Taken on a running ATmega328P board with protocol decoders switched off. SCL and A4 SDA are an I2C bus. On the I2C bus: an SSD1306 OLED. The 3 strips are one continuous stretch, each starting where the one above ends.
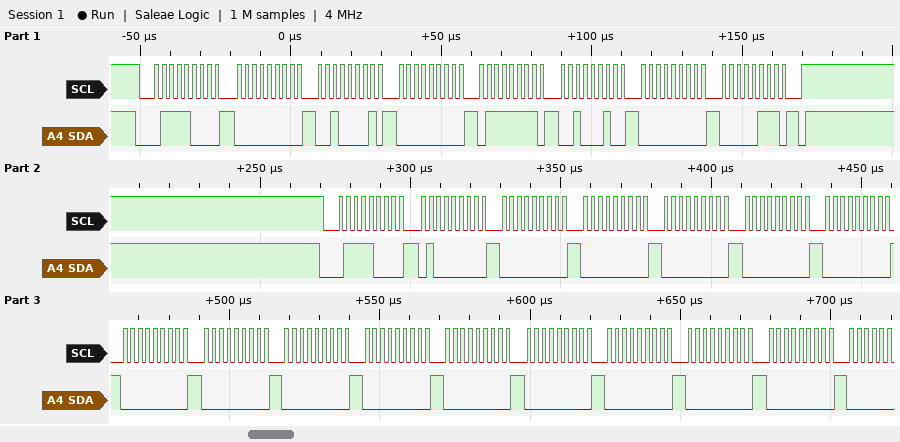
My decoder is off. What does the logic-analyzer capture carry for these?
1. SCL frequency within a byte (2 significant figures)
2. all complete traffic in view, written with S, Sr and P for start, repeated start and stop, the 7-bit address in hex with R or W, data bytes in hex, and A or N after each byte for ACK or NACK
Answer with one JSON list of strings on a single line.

["400 kHz", "S 3CW A 00 A 21 A 00 A 7F A 22 A 00 A 07 A P S 3CW A 40 A 00 A 00 A 00 A 00 A 00 A 00 A 00 A 00 A 00 A 00 A 00 A 00 A 00 A 00 A"]
